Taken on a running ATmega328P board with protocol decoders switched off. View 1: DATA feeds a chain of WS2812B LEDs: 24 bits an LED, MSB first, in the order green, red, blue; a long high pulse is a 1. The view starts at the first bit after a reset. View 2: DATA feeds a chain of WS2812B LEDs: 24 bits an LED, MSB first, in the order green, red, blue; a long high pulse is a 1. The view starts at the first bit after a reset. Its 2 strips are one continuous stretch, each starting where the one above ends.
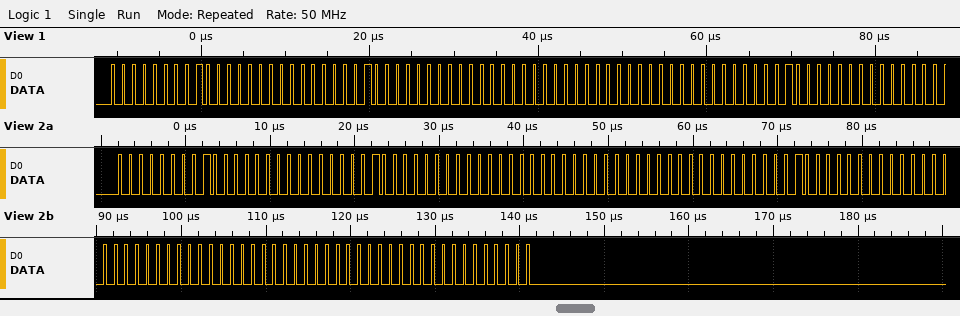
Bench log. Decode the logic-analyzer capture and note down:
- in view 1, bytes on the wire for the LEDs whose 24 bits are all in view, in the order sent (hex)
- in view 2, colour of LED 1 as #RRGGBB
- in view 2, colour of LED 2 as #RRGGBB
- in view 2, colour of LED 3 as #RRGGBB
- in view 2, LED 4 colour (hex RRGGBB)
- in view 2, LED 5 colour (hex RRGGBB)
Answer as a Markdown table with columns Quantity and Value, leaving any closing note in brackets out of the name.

| Quantity | Value |
|---|---|
| in view 1, bytes on the wire for the LEDs whose 24 bits are all in view, in the order sent | 00 80 00 80 00 00 00 00 80 |
| in view 2, colour of LED 1 as #RRGGBB | #800000 |
| in view 2, colour of LED 2 as #RRGGBB | #008000 |
| in view 2, colour of LED 3 as #RRGGBB | #000080 |
| in view 2, LED 4 colour | #000000 |
| in view 2, LED 5 colour | #000000 |
